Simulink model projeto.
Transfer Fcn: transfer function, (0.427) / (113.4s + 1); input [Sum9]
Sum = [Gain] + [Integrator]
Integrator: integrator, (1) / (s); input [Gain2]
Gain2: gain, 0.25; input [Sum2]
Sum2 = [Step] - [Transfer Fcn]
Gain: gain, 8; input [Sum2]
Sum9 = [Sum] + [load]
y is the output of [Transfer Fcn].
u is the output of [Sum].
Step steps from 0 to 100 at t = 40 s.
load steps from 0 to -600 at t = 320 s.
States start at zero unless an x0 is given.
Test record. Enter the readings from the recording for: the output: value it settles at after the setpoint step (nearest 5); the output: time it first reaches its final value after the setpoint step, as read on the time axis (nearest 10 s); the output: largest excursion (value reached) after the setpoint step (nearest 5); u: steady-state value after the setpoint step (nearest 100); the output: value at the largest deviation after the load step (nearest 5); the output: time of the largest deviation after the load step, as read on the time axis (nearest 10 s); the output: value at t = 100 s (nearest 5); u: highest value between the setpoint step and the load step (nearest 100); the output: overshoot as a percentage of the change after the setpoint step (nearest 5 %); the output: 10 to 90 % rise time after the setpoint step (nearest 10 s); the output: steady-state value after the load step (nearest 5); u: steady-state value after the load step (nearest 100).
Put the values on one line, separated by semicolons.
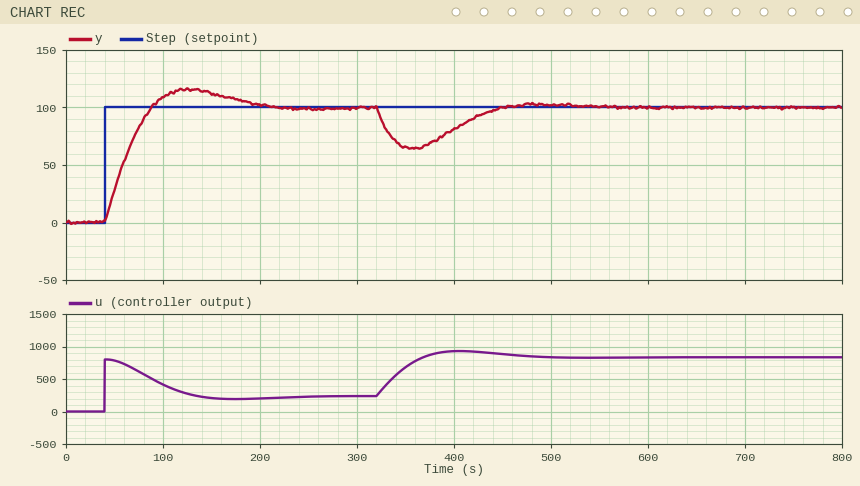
100; 90 s; 115; 200; 65; 360 s; 110; 800; 15 %; 40 s; 100; 800
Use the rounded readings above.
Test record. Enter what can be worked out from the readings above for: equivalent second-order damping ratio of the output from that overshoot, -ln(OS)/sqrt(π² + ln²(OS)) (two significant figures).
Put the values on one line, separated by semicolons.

0.52
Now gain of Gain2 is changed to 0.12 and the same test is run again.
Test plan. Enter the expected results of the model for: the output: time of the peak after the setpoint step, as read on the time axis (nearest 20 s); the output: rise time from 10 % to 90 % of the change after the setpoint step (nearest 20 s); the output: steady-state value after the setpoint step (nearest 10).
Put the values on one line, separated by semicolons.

160 s; 60 s; 100
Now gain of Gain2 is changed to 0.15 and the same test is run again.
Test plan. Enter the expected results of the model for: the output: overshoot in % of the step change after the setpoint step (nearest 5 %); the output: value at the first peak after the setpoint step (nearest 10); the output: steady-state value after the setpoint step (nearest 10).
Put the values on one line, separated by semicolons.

10 %; 110; 100
